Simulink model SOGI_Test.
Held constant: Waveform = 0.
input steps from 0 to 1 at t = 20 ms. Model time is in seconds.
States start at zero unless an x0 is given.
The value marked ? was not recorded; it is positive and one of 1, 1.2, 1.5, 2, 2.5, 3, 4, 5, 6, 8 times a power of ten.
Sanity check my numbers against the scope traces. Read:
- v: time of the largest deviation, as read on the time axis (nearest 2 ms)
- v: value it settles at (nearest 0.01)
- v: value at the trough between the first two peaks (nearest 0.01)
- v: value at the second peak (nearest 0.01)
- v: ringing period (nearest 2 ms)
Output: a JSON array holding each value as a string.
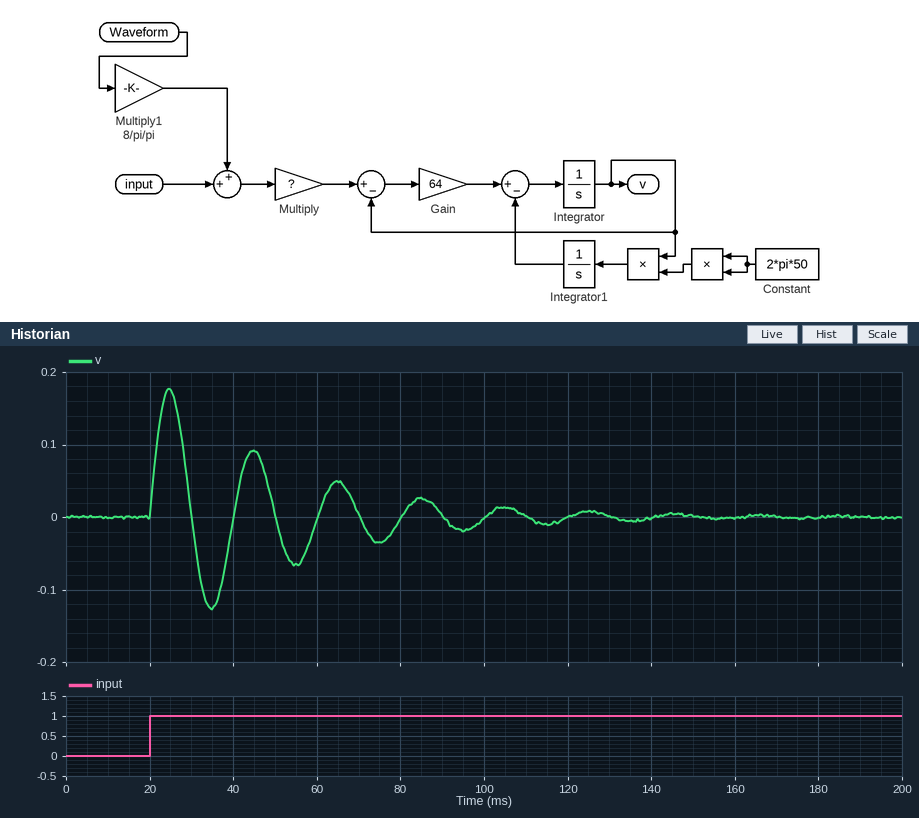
["24 ms", "0.00", "-0.13", "0.09", "20 ms"]
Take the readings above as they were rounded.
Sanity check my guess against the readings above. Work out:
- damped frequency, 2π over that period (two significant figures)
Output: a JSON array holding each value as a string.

["0.31 rad/ms"]
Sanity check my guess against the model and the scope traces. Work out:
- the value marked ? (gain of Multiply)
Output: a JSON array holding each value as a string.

["1"]
